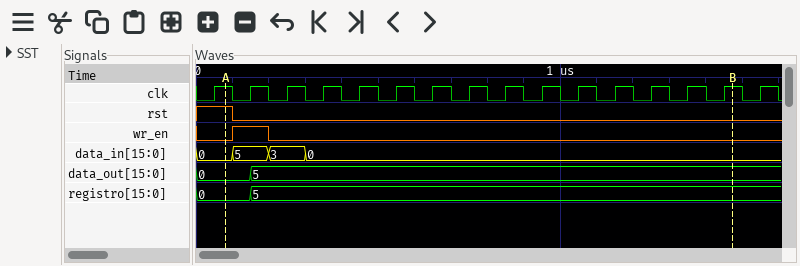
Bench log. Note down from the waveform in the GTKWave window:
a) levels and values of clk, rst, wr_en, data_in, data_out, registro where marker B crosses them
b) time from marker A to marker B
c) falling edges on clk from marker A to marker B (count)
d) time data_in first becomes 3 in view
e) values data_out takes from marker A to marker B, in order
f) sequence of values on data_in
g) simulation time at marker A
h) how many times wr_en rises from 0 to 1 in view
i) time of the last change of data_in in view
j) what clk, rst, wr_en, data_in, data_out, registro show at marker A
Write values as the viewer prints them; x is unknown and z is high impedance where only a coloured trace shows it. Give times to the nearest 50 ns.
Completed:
clk=1, rst=0, wr_en=0, data_in=0, data_out=5, registro=5
1400 ns
14
200 ns
0, 5
0, 5, 3, 0
100 ns
1
300 ns
clk=1, rst=1, wr_en=0, data_in=0, data_out=0, registro=0
